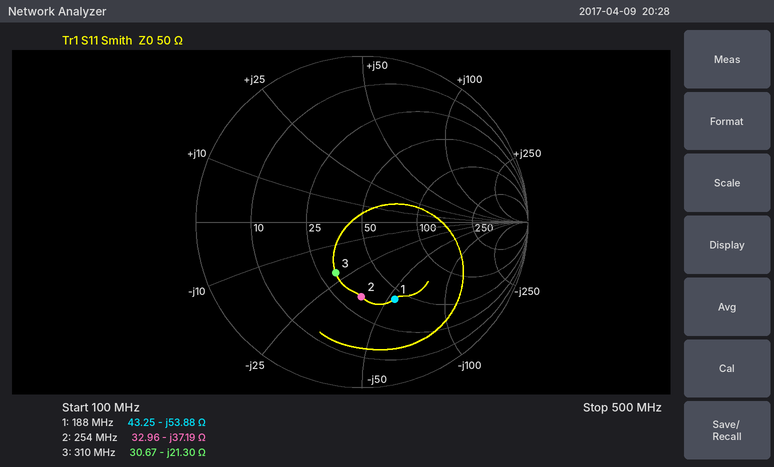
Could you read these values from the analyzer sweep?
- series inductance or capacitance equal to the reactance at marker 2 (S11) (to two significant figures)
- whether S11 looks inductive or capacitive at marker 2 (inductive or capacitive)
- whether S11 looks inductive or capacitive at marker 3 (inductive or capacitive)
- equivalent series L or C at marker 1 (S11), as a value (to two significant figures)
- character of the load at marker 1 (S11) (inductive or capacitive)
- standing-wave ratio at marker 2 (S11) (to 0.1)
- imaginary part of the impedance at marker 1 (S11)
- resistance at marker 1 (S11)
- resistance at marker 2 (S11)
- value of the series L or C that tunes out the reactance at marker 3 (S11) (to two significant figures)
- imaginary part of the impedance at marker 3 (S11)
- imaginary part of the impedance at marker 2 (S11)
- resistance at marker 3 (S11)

17 pF
capacitive
capacitive
16 pF
capacitive
2.6
-53.88 Ω
43.25 Ω
32.96 Ω
11 nH
-21.30 Ω
-37.19 Ω
30.67 Ω
